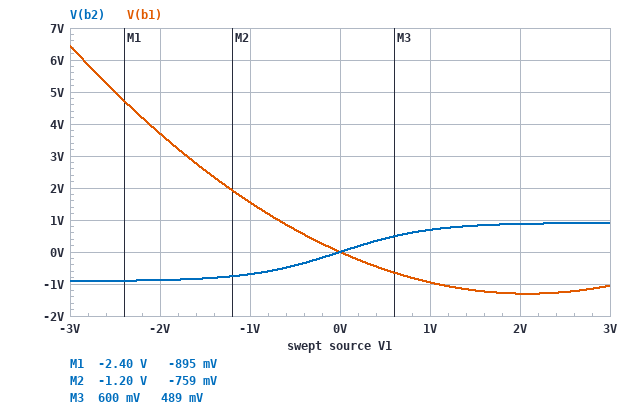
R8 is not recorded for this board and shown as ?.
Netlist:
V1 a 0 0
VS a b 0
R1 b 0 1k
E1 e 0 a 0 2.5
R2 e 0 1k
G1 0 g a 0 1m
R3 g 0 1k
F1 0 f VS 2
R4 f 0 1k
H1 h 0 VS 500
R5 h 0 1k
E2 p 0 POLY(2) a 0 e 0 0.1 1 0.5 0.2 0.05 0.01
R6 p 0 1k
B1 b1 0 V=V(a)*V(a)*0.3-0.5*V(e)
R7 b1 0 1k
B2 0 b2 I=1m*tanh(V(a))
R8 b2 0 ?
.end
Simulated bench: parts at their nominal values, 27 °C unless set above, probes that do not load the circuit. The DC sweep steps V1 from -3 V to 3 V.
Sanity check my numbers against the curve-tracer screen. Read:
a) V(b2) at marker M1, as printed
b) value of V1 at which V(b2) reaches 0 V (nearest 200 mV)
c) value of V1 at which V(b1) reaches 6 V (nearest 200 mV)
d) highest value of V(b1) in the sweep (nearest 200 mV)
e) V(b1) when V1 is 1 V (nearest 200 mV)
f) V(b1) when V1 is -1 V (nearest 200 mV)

-895 mV
0 V
-2.8 V
6.4 V
-1.0 V
1.6 V
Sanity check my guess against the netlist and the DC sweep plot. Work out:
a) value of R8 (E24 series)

910 Ω
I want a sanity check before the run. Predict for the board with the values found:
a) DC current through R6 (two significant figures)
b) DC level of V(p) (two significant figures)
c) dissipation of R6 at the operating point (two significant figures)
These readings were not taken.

100 µA
100 mV
10 µW
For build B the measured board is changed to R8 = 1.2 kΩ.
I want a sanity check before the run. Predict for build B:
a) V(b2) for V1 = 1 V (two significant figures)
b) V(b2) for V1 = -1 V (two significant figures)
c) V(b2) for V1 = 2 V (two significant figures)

910 mV
-910 mV
1.2 V
